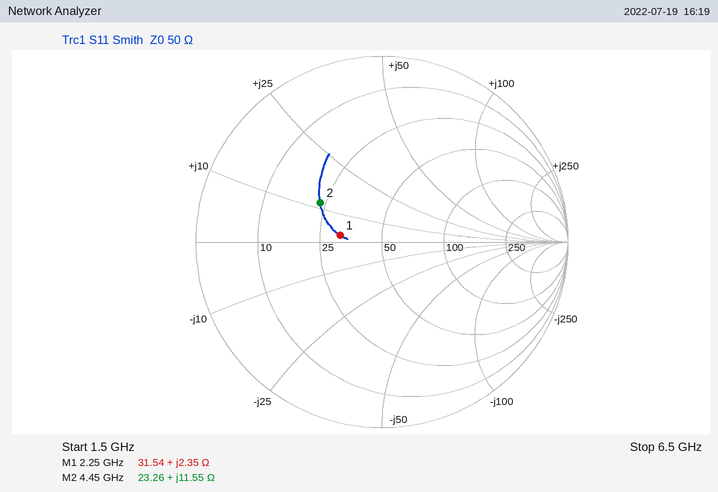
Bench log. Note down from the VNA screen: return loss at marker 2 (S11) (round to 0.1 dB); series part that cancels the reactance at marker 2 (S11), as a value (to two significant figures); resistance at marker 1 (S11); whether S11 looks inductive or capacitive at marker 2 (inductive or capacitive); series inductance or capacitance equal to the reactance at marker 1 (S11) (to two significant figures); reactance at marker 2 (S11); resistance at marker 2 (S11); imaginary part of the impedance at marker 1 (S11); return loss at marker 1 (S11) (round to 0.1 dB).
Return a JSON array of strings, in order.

["8.1 dB", "3.1 pF", "31.54 Ω", "inductive", "170 pH", "+11.55 Ω", "23.26 Ω", "+2.35 Ω", "12.8 dB"]
